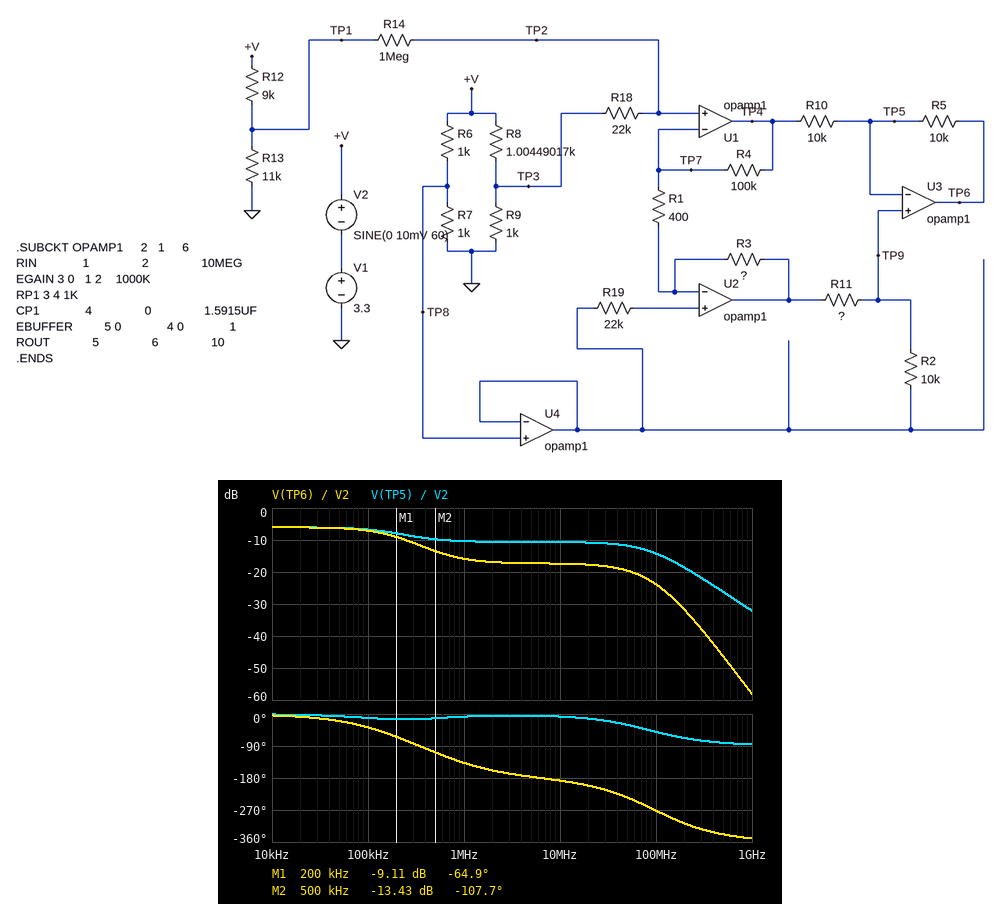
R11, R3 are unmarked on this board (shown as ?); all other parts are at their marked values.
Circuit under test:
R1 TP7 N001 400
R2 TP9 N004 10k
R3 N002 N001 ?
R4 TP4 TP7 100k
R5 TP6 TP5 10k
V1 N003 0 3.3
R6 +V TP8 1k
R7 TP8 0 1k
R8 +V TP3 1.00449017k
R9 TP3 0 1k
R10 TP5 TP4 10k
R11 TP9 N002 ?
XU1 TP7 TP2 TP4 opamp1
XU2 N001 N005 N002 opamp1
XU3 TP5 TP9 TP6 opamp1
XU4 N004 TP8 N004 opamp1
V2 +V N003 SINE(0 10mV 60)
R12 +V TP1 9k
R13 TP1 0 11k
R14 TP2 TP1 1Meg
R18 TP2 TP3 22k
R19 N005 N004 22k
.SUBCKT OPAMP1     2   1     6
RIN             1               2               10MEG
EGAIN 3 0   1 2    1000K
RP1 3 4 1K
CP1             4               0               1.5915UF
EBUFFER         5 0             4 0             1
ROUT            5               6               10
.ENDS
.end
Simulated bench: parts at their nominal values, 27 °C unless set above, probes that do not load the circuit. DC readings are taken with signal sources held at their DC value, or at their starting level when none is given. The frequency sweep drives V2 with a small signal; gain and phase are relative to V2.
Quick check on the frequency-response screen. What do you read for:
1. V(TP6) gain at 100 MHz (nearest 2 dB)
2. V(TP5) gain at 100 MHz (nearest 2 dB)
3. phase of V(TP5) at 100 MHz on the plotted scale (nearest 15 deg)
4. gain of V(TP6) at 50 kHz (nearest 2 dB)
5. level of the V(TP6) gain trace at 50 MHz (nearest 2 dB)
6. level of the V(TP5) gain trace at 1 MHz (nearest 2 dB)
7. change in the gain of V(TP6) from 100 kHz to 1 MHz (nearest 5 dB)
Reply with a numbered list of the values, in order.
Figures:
1. -24 dB
2. -14 dB
3. -45 deg
4. -6 dB
5. -20 dB
6. -10 dB
7. -10 dB
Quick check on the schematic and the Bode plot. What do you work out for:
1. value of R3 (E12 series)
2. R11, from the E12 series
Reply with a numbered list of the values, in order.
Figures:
1. 120 kΩ
2. 3.3 kΩ
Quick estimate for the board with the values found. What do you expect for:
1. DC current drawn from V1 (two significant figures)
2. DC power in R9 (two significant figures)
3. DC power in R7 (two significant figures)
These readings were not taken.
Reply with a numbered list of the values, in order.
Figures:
1. 3.5 mA
2. 2.7 mW
3. 2.7 mW
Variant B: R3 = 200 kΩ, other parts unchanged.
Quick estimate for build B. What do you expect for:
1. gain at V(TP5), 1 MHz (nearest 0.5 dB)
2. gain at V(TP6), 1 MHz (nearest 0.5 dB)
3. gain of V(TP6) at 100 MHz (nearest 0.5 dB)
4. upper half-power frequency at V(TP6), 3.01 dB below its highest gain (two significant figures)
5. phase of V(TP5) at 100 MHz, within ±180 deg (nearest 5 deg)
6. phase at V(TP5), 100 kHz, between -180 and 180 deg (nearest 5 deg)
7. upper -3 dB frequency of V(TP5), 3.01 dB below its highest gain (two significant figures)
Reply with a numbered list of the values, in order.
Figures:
1. -12.0 dB
2. -15.0 dB
3. -23.5 dB
4. 150 kHz
5. -45 deg
6. -15 deg
7. 190 kHz
